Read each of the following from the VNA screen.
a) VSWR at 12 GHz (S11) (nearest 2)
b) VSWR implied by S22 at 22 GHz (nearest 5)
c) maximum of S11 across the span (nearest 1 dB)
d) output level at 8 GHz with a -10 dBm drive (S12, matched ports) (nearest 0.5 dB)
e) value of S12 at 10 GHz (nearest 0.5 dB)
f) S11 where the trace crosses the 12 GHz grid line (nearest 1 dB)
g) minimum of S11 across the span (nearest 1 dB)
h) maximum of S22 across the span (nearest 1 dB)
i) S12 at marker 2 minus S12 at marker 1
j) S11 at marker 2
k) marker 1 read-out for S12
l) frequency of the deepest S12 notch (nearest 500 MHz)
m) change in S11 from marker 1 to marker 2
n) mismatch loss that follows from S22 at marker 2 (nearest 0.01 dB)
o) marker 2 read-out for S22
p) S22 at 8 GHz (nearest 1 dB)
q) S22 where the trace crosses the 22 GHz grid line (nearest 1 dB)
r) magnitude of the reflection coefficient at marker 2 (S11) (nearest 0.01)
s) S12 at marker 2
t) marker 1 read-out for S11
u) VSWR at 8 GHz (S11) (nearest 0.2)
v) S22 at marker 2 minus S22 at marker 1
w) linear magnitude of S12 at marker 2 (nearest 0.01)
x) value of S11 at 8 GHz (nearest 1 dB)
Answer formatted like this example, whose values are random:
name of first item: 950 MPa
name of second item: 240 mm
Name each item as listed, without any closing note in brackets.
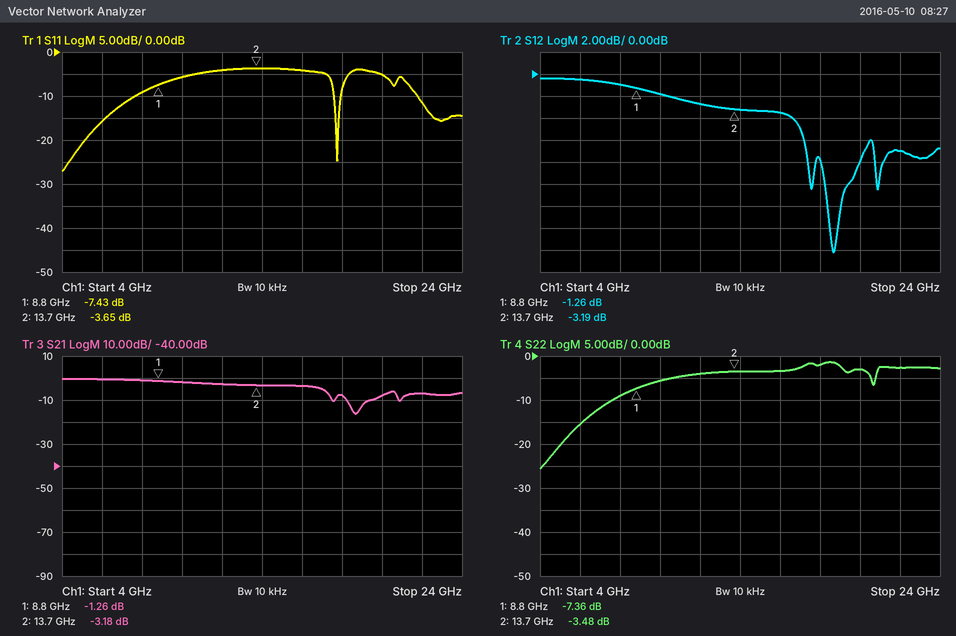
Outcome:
VSWR at 12 GHz (S11): 4
VSWR implied by S22 at 22 GHz: 5
maximum of S11 across the span: -4 dB
output level at 8 GHz with a -10 dBm drive (S12, matched ports): -11.0 dBm
value of S12 at 10 GHz: -2.0 dB
S11 where the trace crosses the 12 GHz grid line: -4 dB
minimum of S11 across the span: -27 dB
maximum of S22 across the span: -1 dB
S12 at marker 2 minus S12 at marker 1: -1.93 dB
S11 at marker 2: -3.65 dB
marker 1 read-out for S12: -1.26 dB
frequency of the deepest S12 notch: 18.5 GHz
change in S11 from marker 1 to marker 2: 3.78 dB
mismatch loss that follows from S22 at marker 2: 2.59 dB
marker 2 read-out for S22: -3.48 dB
S22 at 8 GHz: -9 dB
S22 where the trace crosses the 22 GHz grid line: -3 dB
magnitude of the reflection coefficient at marker 2 (S11): 0.66
S12 at marker 2: -3.19 dB
marker 1 read-out for S11: -7.43 dB
VSWR at 8 GHz (S11): 2.0
S22 at marker 2 minus S22 at marker 1: 3.88 dB
linear magnitude of S12 at marker 2: 0.69
value of S11 at 8 GHz: -9 dB
